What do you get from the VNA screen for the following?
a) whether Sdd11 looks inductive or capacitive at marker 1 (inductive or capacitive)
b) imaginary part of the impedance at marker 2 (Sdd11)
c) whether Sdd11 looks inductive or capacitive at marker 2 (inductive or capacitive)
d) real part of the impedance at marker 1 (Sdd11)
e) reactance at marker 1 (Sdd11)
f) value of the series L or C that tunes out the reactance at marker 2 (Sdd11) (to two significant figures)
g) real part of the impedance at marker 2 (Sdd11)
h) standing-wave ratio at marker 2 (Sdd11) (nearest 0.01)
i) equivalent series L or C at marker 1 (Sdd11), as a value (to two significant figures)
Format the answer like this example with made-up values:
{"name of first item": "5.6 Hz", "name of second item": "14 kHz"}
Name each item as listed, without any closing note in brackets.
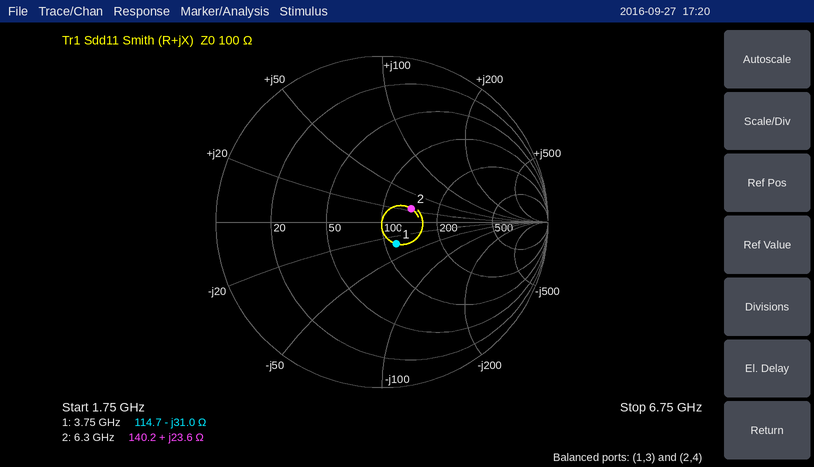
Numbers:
{"whether Sdd11 looks inductive or capacitive at marker 1": "capacitive", "imaginary part of the impedance at marker 2": "+23.6 Ω", "whether Sdd11 looks inductive or capacitive at marker 2": "inductive", "real part of the impedance at marker 1": "114.7 Ω", "reactance at marker 1": "-31.0 Ω", "value of the series L or C that tunes out the reactance at marker 2 (Sdd11)": "1.1 pF", "real part of the impedance at marker 2": "140.2 Ω", "standing-wave ratio at marker 2 (Sdd11)": "1.48", "equivalent series L or C at marker 1 (Sdd11), as a value": "1.4 pF"}
